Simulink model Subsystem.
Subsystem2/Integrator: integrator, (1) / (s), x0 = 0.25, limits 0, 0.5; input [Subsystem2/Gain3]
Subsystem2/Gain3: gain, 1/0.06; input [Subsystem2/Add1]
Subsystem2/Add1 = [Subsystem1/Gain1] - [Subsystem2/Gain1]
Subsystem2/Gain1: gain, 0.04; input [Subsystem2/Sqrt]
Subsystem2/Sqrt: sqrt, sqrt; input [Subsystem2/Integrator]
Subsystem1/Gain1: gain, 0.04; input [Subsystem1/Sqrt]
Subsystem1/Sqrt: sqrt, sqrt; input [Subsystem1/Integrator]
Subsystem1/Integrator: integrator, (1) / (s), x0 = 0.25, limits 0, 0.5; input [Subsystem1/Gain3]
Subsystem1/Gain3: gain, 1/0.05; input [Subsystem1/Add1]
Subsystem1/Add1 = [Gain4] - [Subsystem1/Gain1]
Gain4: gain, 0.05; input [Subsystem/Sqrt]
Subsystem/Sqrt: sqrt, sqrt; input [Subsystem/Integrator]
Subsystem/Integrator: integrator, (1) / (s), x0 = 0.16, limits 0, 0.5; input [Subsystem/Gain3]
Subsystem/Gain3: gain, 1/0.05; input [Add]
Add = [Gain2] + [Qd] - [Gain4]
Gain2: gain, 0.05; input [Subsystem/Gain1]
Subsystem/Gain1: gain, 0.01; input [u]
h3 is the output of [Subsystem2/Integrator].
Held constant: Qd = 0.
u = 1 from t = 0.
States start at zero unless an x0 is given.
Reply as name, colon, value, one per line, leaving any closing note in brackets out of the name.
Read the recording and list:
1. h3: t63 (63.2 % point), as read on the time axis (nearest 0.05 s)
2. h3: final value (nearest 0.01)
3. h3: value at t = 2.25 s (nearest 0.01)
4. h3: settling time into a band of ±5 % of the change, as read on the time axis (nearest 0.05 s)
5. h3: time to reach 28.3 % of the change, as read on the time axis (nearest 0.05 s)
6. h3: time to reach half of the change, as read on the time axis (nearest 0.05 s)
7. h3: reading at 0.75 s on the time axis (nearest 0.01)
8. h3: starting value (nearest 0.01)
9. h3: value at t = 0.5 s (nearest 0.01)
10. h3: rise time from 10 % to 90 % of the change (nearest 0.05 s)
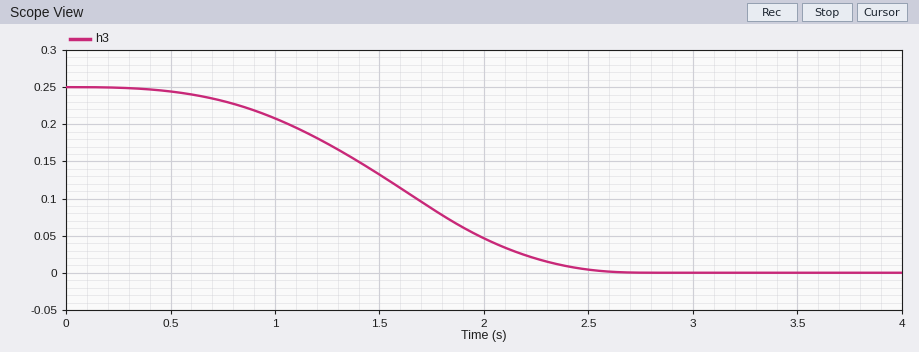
h3: t63 (63.2 % point), as read on the time axis: 1.70 s
h3: final value: 0.00
h3: value at t = 2.25 s: 0.02
h3: settling time into a band of ±5 % of the change, as read on the time axis: 2.35 s
h3: time to reach 28.3 % of the change, as read on the time axis: 1.20 s
h3: time to reach half of the change, as read on the time axis: 1.55 s
h3: reading at 0.75 s on the time axis: 0.23
h3: starting value: 0.25
h3: value at t = 0.5 s: 0.24
h3: rise time from 10 % to 90 % of the change: 1.35 s
